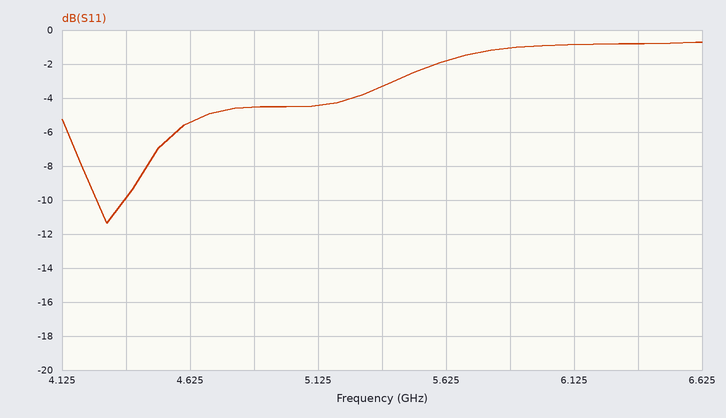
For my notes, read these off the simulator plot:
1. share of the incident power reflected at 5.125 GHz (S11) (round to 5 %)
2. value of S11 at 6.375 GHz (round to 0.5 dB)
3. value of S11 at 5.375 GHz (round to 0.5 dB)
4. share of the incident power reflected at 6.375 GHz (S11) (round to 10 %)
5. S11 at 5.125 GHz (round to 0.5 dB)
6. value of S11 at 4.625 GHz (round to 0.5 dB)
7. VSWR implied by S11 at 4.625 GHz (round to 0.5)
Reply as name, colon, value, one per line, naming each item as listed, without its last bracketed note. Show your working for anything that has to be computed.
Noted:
share of the incident power reflected at 5.125 GHz (S11): 10^(-4.5/10) ≈ 35 %
value of S11 at 6.375 GHz: -1.0 dB
value of S11 at 5.375 GHz: -3.5 dB
share of the incident power reflected at 6.375 GHz (S11): 10^(-1/10) ≈ 79.4 %, so 80 % to the nearest 10 %
S11 at 5.125 GHz: -4.5 dB
value of S11 at 4.625 GHz: -5.5 dB
VSWR implied by S11 at 4.625 GHz: |Γ| = 10^(-5.5/20) = 0.5309; VSWR = (1 + 0.5309)/(1 − 0.5309) ≈ 3.26, so 3.5 to the nearest 0.5
